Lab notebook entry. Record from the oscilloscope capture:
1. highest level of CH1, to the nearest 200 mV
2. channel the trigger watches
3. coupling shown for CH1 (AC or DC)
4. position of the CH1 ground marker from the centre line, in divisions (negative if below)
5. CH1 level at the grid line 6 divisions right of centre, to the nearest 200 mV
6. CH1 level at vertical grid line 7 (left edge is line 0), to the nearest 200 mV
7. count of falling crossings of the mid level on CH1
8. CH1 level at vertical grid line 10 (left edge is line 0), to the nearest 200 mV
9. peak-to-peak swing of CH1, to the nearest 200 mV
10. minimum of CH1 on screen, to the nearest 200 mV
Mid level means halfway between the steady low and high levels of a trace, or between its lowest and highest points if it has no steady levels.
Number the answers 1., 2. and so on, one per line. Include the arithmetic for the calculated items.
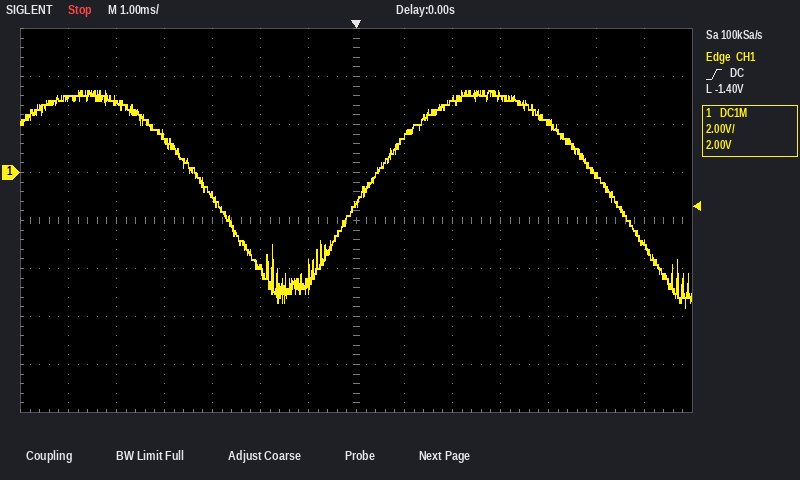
1. 3.4 V
2. CH1
3. DC
4. +1.0 div
5. -3.0 V
6. -1.2 V
7. 2
8. 3.2 V
9. 3.4 V − (-5.6 V) = 9.0 V
10. -5.6 V
